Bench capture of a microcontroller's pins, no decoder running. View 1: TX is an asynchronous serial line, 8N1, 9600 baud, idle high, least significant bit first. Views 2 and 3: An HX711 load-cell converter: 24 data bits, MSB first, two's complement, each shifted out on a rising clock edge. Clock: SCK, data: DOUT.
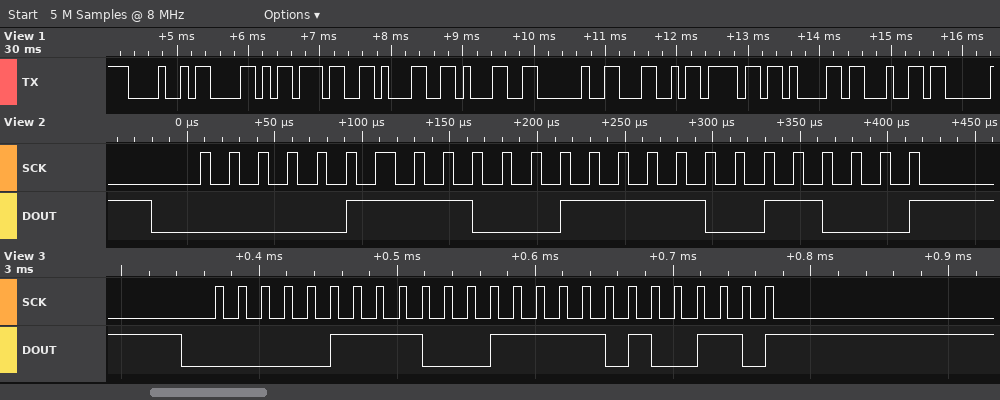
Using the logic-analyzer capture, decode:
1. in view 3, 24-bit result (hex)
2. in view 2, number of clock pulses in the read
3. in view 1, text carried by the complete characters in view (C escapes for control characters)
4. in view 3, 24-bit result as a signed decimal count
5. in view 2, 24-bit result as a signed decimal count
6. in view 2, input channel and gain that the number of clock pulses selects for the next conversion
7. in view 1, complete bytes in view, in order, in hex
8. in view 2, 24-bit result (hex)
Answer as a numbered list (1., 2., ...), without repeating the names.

1. 0x078FA6
2. 25
3. "HX711 Load"
4. 495526
5. 495512
6. channel A, gain 128
7. 48 58 37 31 31 20 4C 6F 61 64
8. 0x078F98
